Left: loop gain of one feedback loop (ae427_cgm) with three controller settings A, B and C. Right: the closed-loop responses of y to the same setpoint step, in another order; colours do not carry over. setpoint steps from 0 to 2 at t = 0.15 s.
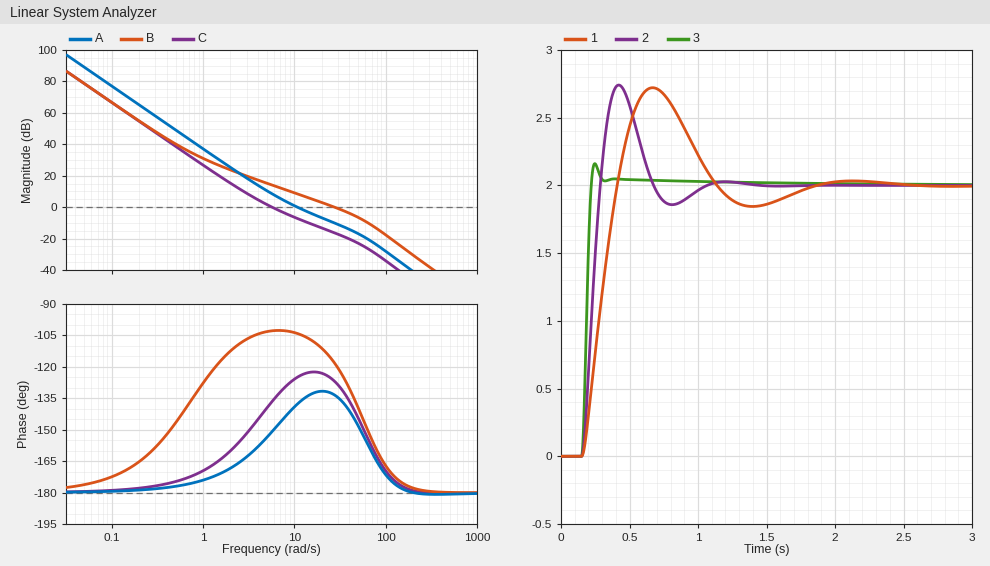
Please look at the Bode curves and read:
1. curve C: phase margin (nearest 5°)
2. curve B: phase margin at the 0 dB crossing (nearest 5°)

45°
60°
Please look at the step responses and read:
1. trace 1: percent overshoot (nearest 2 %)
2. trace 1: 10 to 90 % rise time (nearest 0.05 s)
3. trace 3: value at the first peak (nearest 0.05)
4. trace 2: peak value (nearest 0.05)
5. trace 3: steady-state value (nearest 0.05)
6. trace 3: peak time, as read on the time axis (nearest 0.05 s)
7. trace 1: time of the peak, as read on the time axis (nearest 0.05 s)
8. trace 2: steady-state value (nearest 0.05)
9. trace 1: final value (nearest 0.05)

36 %
0.20 s
2.15
2.75
2.00
0.25 s
0.65 s
2.00
2.00
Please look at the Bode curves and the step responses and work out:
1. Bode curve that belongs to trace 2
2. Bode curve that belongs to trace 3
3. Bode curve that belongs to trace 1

A
B
C
